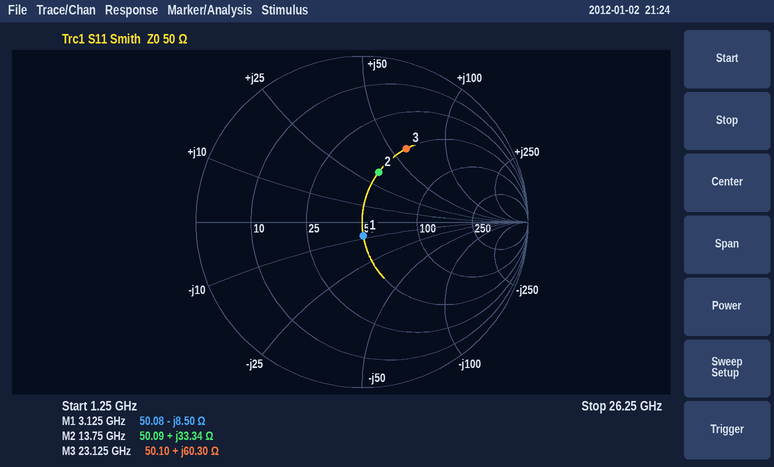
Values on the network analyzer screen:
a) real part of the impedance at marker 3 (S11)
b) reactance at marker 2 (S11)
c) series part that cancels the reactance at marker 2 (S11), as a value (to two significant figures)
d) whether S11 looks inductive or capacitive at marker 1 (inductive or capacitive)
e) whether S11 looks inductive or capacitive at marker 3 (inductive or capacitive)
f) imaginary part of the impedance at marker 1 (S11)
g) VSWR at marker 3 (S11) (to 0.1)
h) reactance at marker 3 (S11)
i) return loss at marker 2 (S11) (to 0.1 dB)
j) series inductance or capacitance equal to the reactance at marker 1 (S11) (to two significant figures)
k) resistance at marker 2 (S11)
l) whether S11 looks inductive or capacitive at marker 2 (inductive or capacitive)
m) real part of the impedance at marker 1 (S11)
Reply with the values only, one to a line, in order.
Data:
50.10 Ω
+33.34 Ω
350 fF
capacitive
inductive
-8.50 Ω
3.1
+60.30 Ω
10.0 dB
6.0 pF
50.09 Ω
inductive
50.08 Ω
